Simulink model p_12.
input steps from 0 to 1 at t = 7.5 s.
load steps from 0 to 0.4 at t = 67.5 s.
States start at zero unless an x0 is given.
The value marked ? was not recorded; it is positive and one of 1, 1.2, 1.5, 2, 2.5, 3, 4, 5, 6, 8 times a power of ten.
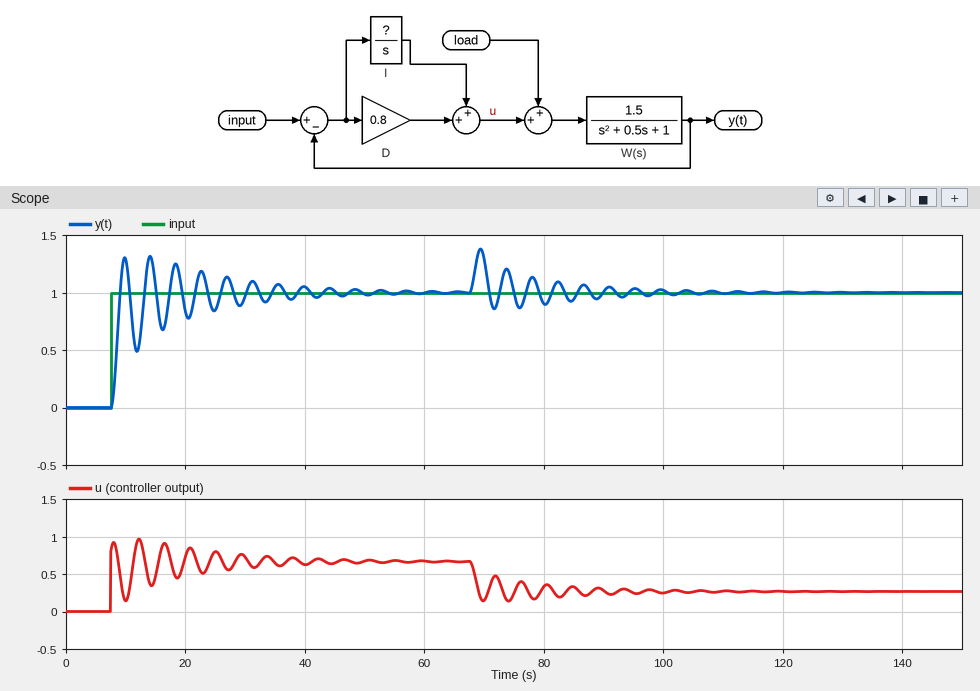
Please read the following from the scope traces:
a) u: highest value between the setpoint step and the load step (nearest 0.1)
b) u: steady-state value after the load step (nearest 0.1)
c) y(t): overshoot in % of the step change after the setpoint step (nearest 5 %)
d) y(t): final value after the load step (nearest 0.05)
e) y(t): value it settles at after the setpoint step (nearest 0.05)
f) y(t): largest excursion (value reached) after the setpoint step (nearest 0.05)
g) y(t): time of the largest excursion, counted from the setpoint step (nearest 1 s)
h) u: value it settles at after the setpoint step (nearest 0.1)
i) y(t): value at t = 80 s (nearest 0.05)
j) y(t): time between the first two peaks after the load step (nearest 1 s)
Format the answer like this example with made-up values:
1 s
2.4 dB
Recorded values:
1.0
0.3
30 %
1.00
1.00
1.30
7 s
0.7
0.90
4 s
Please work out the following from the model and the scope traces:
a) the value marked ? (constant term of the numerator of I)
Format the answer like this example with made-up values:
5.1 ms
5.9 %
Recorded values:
0.5
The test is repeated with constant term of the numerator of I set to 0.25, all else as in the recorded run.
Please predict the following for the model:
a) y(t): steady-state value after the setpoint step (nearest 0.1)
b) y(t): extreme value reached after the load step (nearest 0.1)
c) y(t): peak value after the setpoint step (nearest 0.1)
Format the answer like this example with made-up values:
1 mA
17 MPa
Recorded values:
1.0
1.4
1.1
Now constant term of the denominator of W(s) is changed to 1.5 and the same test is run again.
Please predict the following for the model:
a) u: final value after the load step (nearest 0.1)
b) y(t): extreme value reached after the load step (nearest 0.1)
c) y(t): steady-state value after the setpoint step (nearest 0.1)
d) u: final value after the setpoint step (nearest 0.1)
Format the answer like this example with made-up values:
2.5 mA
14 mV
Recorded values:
0.6
1.3
1.0
1.0
